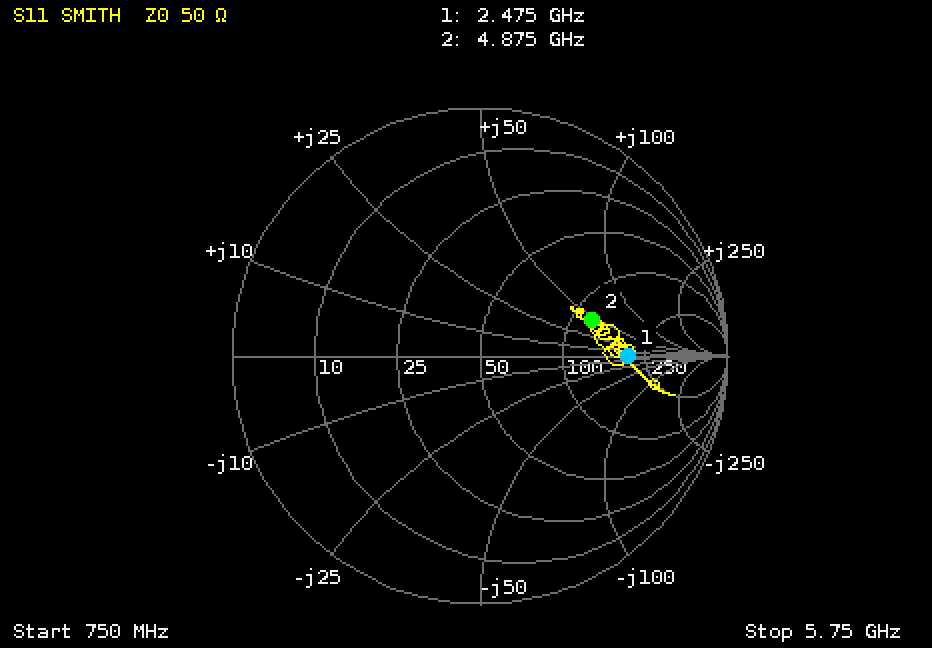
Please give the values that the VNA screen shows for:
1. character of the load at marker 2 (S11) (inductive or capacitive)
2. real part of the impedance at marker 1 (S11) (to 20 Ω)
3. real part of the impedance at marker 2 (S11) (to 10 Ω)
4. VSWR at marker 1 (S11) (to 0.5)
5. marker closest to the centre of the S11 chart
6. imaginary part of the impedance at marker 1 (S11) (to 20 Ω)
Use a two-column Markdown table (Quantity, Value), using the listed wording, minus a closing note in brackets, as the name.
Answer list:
| Quantity | Value |
|---|---|
| character of the load at marker 2 (S11) | inductive |
| real part of the impedance at marker 1 (S11) | 200 Ω |
| real part of the impedance at marker 2 (S11) | 120 Ω |
| VSWR at marker 1 (S11) | 4.0 |
| marker closest to the centre of the S11 chart | marker 2 |
| imaginary part of the impedance at marker 1 (S11) | 0 Ω |
